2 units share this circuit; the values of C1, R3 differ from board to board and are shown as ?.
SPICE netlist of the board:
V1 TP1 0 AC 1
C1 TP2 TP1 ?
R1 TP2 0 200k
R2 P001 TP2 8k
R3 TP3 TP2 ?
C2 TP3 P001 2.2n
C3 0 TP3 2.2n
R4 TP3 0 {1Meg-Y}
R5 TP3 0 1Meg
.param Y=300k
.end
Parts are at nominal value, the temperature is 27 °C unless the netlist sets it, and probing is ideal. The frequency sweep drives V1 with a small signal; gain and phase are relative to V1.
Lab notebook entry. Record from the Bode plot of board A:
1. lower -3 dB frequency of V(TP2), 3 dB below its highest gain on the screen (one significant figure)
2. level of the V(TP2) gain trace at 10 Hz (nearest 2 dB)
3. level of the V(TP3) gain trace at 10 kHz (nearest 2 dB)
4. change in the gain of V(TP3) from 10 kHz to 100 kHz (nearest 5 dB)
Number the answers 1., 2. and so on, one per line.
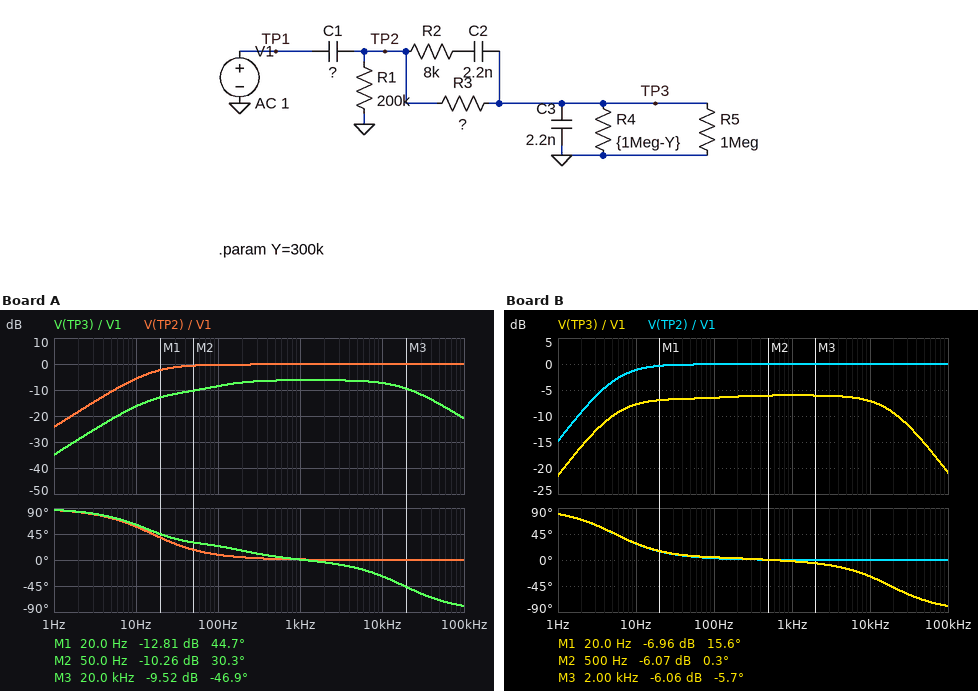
1. 20 Hz
2. -6 dB
3. -8 dB
4. -15 dB
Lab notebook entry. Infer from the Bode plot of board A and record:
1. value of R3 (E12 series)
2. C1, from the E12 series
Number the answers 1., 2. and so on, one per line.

1. 1 MΩ
2. 56 nF
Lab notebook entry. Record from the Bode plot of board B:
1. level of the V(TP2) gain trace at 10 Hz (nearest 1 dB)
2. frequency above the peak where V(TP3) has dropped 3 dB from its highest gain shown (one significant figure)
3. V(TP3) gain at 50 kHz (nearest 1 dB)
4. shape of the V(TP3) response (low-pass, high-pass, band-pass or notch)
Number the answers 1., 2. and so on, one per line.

1. -1 dB
2. 20 kHz
3. -15 dB
4. band-pass
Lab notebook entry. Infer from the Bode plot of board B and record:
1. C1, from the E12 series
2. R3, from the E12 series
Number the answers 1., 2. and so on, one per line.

1. 180 nF
2. 470 kΩ
